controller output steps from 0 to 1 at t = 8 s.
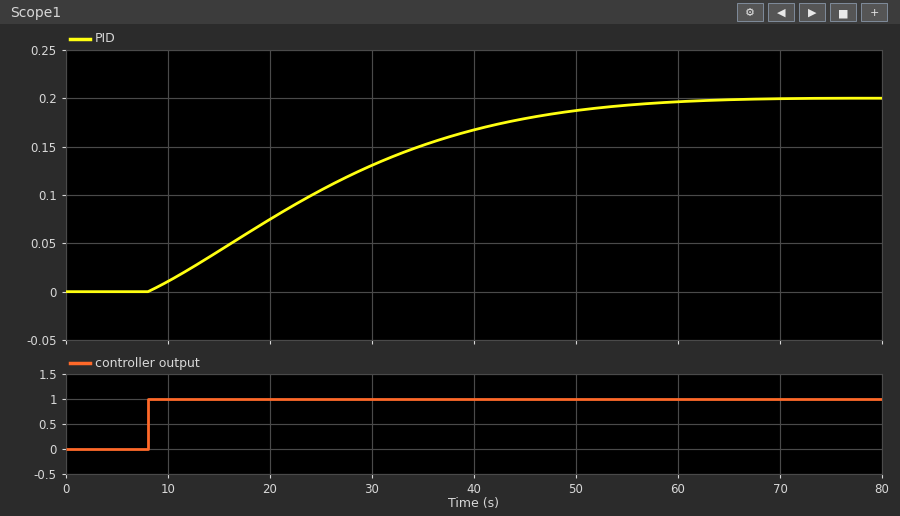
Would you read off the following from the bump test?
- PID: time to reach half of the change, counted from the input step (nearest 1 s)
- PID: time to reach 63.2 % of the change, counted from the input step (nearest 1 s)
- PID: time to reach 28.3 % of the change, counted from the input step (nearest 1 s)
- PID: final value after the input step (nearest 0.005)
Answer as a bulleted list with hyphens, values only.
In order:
- 16 s
- 21 s
- 9 s
- 0.200
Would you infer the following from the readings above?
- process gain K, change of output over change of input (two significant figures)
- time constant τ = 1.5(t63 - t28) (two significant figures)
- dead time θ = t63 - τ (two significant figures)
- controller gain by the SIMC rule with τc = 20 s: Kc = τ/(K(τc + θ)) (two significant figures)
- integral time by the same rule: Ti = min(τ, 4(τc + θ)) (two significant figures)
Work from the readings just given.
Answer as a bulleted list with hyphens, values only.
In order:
- 0.20
- 18 s
- 3.0 s
- 3.9
- 18 s
